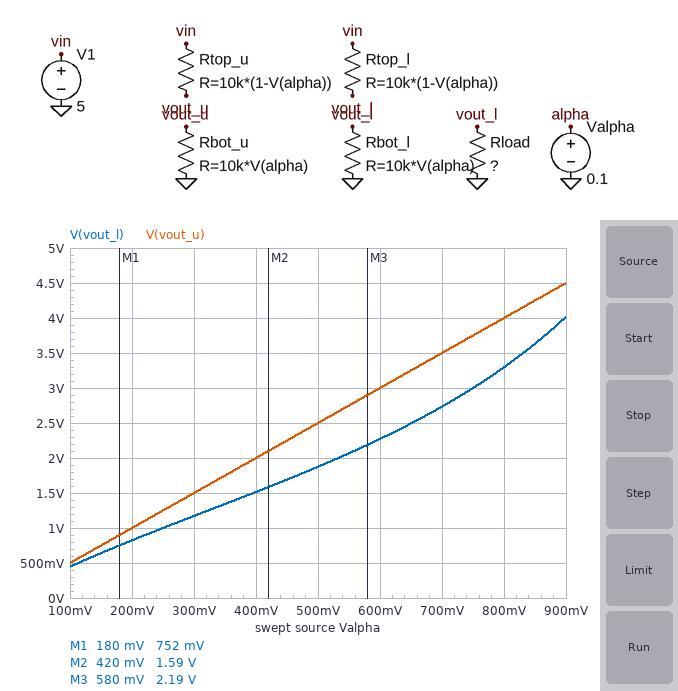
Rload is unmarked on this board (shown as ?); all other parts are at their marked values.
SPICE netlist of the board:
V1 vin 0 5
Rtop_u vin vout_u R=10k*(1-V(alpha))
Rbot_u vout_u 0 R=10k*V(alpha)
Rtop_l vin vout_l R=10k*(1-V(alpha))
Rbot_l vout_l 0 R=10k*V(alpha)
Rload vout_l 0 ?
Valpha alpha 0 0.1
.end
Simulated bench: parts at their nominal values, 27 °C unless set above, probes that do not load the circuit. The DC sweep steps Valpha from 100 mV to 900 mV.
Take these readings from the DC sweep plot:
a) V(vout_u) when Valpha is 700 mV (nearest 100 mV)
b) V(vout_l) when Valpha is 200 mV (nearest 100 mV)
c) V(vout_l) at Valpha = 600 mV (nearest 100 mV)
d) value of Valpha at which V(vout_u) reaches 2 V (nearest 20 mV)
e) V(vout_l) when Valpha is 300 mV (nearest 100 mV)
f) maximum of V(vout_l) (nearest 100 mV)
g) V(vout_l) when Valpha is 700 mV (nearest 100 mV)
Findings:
3.5 V
800 mV
2.3 V
400 mV
1.2 V
4.0 V
2.7 V
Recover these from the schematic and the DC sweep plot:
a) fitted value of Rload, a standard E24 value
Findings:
7.5 kΩ
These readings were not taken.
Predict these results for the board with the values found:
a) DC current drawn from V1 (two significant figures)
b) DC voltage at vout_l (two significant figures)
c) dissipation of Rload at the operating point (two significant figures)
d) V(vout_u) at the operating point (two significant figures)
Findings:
1.0 mA
450 mV
27 µW
500 mV
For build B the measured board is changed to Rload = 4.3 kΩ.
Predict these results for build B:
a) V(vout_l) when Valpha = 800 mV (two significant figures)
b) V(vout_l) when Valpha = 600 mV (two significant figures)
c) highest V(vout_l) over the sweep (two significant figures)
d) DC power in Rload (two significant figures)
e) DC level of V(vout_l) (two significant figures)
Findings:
2.9 V
1.9 V
3.7 V
40 µW
410 mV
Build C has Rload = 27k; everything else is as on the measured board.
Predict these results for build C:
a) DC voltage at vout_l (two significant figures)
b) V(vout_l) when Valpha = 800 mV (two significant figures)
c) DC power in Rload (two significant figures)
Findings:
480 mV
3.8 V
8.7 µW
